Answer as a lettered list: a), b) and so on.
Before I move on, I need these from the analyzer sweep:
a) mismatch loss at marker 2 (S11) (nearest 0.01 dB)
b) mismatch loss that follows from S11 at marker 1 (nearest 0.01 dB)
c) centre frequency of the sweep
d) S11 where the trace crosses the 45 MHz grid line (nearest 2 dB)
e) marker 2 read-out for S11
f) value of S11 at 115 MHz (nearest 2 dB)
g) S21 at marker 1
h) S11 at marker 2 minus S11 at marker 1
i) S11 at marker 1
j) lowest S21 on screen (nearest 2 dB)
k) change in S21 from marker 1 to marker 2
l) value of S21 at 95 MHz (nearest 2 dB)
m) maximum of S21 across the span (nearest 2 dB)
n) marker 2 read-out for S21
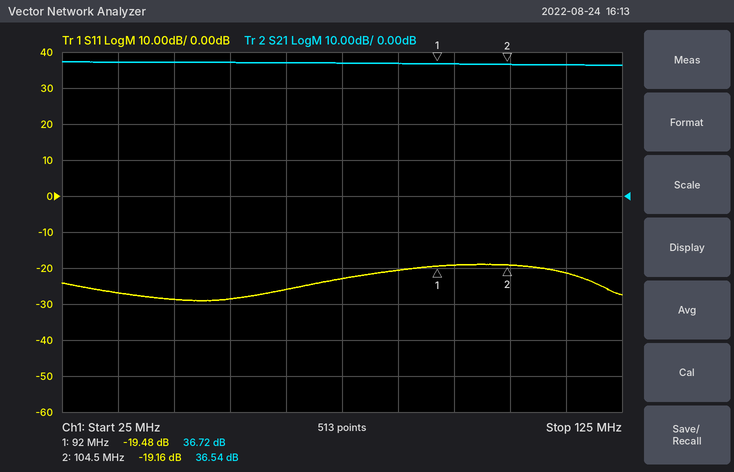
a) 0.05 dB
b) 0.05 dB
c) 75 MHz
d) -28 dB
e) -19.16 dB
f) -22 dB
g) 36.72 dB
h) 0.32 dB
i) -19.48 dB
j) 36 dB
k) -0.18 dB
l) 36 dB
m) 38 dB
n) 36.54 dB
